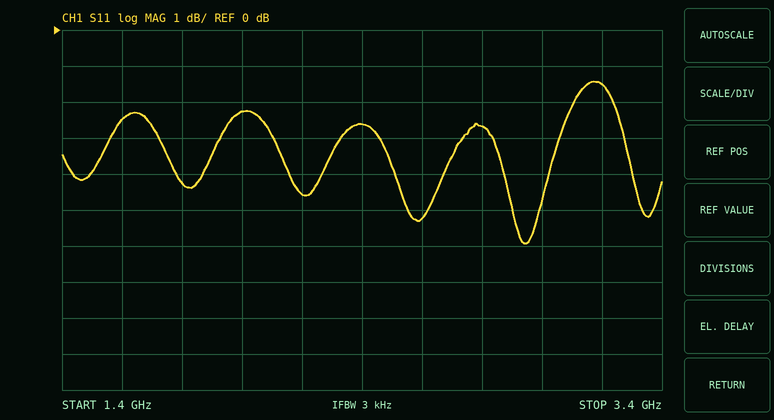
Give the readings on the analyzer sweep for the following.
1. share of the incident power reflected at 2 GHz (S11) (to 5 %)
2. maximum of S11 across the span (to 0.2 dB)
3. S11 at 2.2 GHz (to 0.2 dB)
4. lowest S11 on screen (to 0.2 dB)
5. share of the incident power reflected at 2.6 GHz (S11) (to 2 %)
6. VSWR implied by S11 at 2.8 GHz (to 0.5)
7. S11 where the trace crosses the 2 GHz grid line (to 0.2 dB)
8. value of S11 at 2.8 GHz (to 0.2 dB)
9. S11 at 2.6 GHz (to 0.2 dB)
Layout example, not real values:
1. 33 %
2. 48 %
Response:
1. 60 %
2. -1.4 dB
3. -4.6 dB
4. -6.0 dB
5. 30 %
6. 6.5
7. -2.2 dB
8. -2.6 dB
9. -5.2 dB
